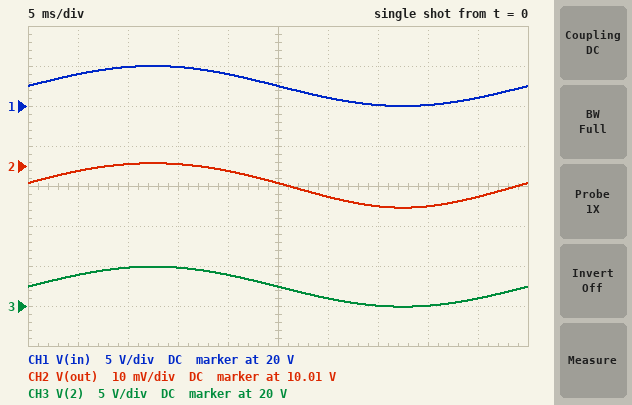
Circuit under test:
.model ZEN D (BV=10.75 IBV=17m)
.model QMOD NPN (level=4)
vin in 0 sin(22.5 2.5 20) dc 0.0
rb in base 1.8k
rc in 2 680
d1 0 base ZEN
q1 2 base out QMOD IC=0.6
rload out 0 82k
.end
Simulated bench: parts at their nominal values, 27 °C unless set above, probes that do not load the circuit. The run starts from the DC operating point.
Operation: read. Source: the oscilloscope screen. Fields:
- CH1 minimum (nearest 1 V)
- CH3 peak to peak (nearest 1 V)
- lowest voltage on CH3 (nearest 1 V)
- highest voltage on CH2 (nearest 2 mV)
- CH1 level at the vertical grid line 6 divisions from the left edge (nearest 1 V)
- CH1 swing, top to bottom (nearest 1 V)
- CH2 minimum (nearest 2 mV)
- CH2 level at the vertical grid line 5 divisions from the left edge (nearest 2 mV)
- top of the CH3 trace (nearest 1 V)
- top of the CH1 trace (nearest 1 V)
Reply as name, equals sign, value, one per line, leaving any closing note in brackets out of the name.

CH1 minimum = 20 V
CH3 peak to peak = 5 V
lowest voltage on CH3 = 20 V
highest voltage on CH2 = 10.010 V
CH1 level at the vertical grid line 6 divisions from the left edge = 21 V
CH1 swing, top to bottom = 5 V
CH2 minimum = 10.000 V
CH2 level at the vertical grid line 5 divisions from the left edge = 10.006 V
top of the CH3 trace = 25 V
top of the CH1 trace = 25 V
